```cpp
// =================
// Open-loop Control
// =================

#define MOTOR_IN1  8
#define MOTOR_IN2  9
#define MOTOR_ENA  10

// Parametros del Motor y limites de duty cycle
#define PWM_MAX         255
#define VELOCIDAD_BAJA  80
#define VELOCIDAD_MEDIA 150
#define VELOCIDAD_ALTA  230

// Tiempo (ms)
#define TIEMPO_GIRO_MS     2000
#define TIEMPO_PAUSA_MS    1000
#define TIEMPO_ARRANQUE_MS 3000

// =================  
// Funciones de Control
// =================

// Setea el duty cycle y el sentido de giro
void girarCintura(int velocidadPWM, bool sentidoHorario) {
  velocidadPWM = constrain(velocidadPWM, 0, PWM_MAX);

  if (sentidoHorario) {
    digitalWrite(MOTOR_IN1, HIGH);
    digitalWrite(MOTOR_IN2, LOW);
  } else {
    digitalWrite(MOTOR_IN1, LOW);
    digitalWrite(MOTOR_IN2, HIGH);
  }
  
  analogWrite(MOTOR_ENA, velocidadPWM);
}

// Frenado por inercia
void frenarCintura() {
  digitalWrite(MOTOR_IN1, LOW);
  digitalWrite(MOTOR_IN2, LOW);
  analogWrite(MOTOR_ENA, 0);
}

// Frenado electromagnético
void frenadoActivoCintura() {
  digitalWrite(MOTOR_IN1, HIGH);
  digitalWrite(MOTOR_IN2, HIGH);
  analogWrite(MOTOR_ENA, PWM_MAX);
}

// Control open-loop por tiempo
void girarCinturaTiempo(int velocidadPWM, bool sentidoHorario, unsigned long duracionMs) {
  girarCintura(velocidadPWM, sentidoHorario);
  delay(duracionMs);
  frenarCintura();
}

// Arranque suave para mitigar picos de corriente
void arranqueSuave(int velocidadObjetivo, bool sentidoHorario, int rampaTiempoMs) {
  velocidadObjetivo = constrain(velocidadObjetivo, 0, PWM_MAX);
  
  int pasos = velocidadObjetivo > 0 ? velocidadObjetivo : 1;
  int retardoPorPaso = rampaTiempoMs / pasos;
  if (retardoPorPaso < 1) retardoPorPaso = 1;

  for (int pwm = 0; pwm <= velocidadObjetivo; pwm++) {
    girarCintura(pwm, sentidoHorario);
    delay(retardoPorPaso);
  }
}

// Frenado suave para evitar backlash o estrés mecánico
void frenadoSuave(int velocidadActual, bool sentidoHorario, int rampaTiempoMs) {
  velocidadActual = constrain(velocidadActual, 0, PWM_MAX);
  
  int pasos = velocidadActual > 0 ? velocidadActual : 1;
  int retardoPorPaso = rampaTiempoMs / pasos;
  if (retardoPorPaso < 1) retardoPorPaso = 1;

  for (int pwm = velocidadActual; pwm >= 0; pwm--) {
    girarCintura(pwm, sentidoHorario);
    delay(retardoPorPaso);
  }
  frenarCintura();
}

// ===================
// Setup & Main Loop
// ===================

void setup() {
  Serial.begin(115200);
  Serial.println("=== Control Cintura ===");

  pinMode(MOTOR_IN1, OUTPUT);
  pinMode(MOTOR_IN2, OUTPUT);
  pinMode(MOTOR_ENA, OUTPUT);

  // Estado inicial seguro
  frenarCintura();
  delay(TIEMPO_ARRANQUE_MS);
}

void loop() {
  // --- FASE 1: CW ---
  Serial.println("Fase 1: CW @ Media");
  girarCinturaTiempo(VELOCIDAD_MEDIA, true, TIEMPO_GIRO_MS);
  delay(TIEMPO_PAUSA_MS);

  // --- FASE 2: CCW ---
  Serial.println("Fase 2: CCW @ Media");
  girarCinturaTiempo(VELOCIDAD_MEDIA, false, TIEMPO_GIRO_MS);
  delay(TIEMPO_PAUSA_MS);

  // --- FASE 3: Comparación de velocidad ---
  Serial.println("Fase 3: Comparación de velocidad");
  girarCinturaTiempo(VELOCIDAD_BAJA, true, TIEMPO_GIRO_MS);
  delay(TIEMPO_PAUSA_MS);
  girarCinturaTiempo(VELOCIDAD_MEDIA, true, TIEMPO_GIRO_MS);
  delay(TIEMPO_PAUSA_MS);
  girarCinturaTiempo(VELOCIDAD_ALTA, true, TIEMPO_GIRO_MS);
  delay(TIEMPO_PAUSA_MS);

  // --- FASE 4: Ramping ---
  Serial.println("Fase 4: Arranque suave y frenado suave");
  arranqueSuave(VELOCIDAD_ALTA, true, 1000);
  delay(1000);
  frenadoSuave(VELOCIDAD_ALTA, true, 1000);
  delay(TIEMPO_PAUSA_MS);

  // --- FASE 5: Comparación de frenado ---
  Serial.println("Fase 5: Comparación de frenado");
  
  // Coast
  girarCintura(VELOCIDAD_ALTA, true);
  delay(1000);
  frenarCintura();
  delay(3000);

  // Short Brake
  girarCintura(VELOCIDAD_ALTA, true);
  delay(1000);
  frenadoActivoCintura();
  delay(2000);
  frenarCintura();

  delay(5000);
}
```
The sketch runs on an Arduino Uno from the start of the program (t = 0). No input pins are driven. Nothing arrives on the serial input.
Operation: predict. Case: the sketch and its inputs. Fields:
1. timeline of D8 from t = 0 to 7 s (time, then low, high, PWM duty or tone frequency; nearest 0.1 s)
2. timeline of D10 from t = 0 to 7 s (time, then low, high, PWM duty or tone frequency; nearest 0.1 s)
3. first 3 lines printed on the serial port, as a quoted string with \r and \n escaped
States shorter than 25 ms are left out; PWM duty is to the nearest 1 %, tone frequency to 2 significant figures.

0 s low; 3 s high; 5 s low
0 s low; 3 s PWM 59 %; 5 s low; 6 s PWM 59 %
"=== Control Cintura ===\r\nFase 1: CW @ Media\r\nFase 2: CCW @ Media\r\n"
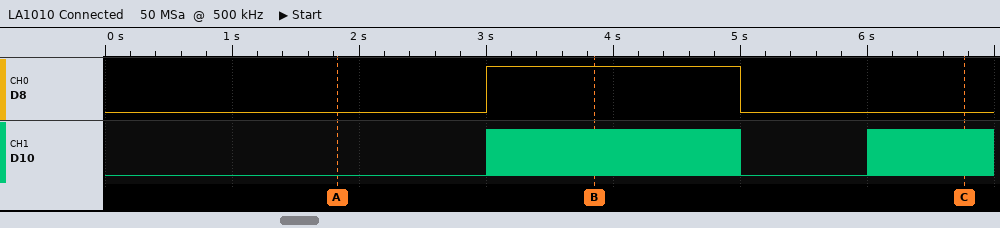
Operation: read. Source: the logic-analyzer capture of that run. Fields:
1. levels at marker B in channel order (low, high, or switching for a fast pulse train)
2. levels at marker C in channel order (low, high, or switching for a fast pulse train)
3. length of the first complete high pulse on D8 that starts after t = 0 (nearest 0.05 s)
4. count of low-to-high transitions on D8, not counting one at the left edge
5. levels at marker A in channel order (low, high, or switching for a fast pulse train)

D8 high, D10 switching
D8 low, D10 switching
2.00 s
1
D8 low, D10 low
